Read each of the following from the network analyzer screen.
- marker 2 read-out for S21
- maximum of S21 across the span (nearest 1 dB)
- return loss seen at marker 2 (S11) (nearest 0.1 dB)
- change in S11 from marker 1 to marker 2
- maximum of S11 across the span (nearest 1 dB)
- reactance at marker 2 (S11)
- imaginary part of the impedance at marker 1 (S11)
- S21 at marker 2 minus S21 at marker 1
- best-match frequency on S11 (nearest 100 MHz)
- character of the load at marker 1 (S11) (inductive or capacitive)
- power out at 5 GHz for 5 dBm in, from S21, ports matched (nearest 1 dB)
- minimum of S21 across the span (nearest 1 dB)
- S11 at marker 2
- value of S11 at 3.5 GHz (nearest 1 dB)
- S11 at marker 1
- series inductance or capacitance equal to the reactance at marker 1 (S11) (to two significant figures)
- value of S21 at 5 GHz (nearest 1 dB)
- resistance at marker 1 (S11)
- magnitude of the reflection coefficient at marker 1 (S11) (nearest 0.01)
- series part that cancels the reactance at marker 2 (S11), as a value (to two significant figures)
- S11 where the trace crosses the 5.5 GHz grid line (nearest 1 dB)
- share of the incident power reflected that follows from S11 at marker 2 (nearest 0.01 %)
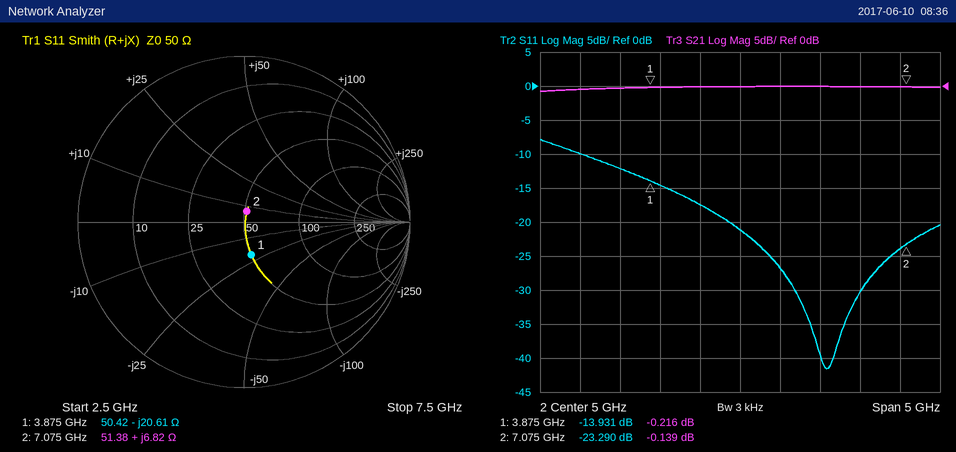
-0.139 dB
0 dB
23.3 dB
-9.359 dB
-8 dB
+6.82 Ω
-20.61 Ω
0.077 dB
6.1 GHz
capacitive
5 dBm
-1 dB
-23.290 dB
-12 dB
-13.931 dB
2.0 pF
0 dB
50.42 Ω
0.20
3.3 pF
-27 dB
0.47 %
